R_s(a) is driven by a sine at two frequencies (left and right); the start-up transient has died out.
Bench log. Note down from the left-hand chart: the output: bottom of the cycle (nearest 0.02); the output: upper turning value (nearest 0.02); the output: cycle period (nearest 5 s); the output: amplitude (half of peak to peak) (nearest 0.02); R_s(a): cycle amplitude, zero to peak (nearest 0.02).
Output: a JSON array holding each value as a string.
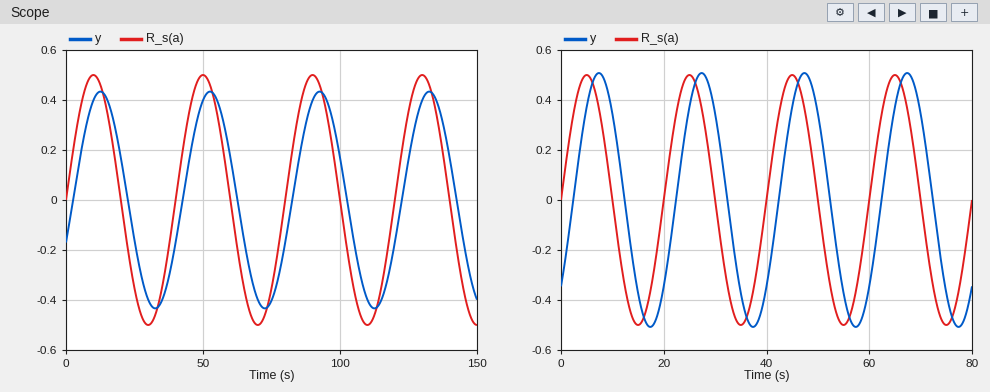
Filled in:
["-0.44", "0.44", "40 s", "0.44", "0.50"]
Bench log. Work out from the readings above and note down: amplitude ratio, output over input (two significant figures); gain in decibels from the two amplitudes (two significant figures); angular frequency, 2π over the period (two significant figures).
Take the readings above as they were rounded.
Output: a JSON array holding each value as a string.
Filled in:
["0.88", "-1.1 dB", "0.16 rad/s"]
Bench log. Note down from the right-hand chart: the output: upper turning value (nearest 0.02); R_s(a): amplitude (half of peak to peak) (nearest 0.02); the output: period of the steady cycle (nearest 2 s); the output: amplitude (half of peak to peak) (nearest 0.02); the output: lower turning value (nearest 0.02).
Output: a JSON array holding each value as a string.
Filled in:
["0.50", "0.50", "20 s", "0.50", "-0.50"]
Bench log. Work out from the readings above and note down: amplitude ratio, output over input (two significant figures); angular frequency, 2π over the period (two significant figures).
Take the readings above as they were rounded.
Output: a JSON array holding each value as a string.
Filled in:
["1.0", "0.31 rad/s"]
